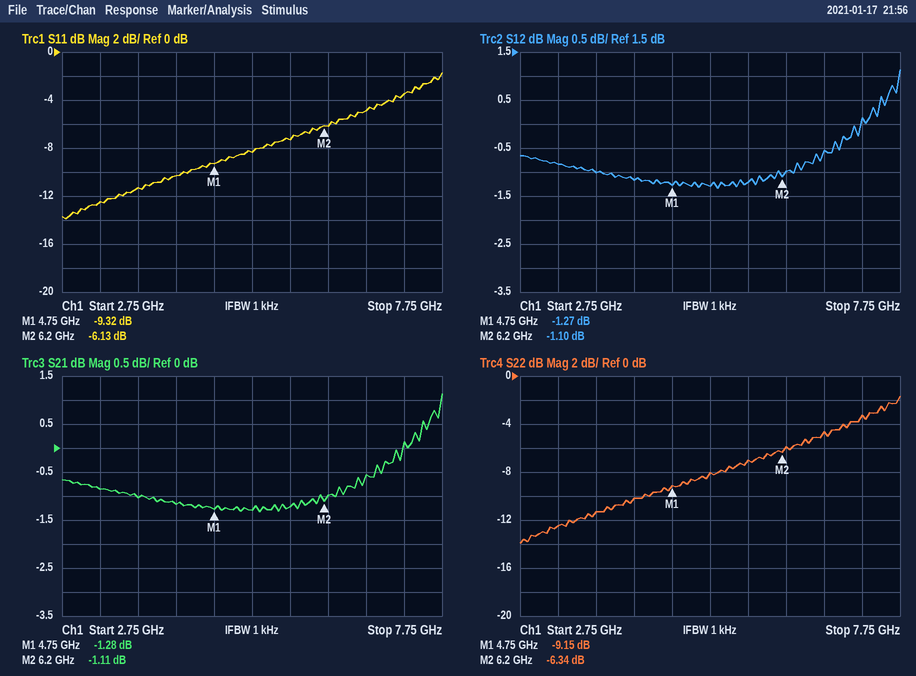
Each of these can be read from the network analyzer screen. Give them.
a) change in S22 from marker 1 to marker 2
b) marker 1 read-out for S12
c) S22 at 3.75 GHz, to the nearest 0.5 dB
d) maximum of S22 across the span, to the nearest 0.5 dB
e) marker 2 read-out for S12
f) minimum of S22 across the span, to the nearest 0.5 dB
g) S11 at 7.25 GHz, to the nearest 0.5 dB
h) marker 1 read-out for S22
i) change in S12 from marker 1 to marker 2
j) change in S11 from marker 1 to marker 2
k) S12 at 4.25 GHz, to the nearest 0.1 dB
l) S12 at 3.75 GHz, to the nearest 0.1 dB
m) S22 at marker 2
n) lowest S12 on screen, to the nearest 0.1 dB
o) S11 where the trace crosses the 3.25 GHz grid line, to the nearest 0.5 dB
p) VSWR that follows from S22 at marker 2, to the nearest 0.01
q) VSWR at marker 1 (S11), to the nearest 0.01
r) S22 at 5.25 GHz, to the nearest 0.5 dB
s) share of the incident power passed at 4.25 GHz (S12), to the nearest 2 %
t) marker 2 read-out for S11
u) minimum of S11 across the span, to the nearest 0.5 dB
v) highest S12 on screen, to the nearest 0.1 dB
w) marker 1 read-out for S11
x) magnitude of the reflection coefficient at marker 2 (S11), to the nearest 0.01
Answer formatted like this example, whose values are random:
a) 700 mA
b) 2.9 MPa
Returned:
a) 2.81 dB
b) -1.27 dB
c) -11.5 dB
d) -1.5 dB
e) -1.10 dB
f) -14.0 dB
g) -3.5 dB
h) -9.15 dB
i) 0.17 dB
j) 3.19 dB
k) -1.2 dB
l) -1.0 dB
m) -6.34 dB
n) -1.3 dB
o) -12.5 dB
p) 2.86
q) 2.04
r) -8.0 dB
s) 76 %
t) -6.13 dB
u) -14.0 dB
v) 1.1 dB
w) -9.32 dB
x) 0.49
